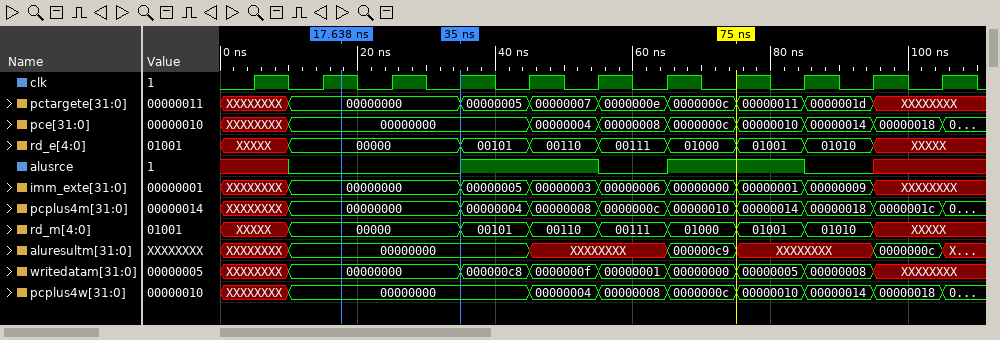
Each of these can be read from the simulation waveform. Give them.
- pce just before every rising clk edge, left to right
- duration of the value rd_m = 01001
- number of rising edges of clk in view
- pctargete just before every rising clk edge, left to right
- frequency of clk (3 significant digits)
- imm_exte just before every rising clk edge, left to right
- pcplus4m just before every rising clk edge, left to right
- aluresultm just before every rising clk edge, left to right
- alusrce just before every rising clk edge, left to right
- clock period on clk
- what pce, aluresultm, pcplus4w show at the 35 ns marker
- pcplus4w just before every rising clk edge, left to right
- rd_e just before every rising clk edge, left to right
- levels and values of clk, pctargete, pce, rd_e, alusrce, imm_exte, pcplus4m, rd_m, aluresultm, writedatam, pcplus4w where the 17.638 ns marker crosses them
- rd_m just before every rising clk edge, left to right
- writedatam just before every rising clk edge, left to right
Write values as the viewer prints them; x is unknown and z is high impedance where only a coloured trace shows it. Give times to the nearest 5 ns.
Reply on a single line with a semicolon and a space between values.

XXXXXXXX, 00000000, 00000000, 00000000, 00000000, 00000004, 00000008, 0000000c, 00000010, 00000014, 00000018; 10 ns; 11; XXXXXXXX, 00000000, 00000000, 00000000, 00000005, 00000007, 0000000e, 0000000c, 00000011, 0000001d, XXXXXXXX; 100 MHz; XXXXXXXX, 00000000, 00000000, 00000000, 00000005, 00000003, 00000006, 00000000, 00000001, 00000009, XXXXXXXX; XXXXXXXX, 00000000, 00000000, 00000000, 00000004, 00000008, 0000000c, 00000010, 00000014, 00000018, 0000001c; XXXXXXXX, 00000000, 00000000, 00000000, 00000000, XXXXXXXX, XXXXXXXX, 000000c9, XXXXXXXX, XXXXXXXX, 0000000c; x 0 0 0 1 1 0 1 1 0 x; 10 ns; pce=00000000, aluresultm=00000000, pcplus4w=00000000; XXXXXXXX, 00000000, 00000000, 00000000, 00000000, 00000004, 00000008, 0000000c, 00000010, 00000014, 00000018; XXXXX, 00000, 00000, 00000, 00101, 00110, 00111, 01000, 01001, 01010, XXXXX; clk=1, pctargete=00000000, pce=00000000, rd_e=00000, alusrce=0, imm_exte=00000000, pcplus4m=00000000, rd_m=00000, aluresultm=00000000, writedatam=00000000, pcplus4w=00000000; XXXXX, 00000, 00000, 00000, 00101, 00110, 00111, 01000, 01001, 01010, XXXXX; XXXXXXXX, 00000000, 00000000, 00000000, 000000c8, 0000000f, 00000001, 00000000, 00000005, 00000008, XXXXXXXX
